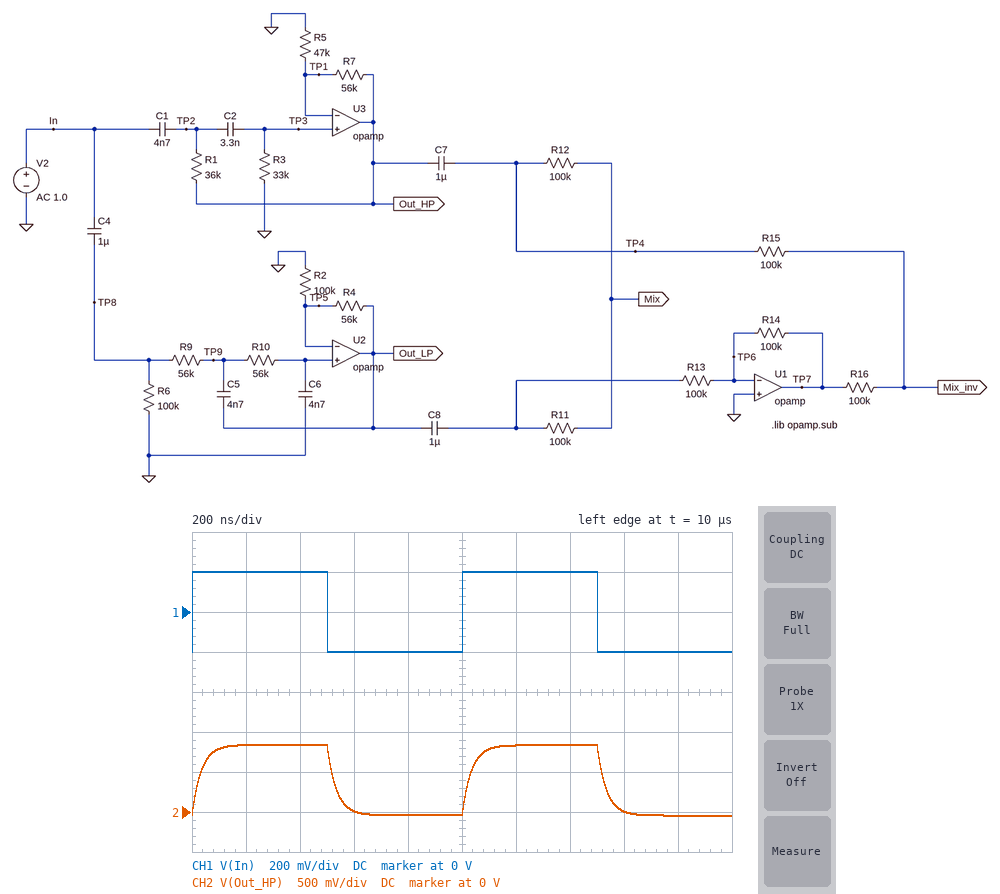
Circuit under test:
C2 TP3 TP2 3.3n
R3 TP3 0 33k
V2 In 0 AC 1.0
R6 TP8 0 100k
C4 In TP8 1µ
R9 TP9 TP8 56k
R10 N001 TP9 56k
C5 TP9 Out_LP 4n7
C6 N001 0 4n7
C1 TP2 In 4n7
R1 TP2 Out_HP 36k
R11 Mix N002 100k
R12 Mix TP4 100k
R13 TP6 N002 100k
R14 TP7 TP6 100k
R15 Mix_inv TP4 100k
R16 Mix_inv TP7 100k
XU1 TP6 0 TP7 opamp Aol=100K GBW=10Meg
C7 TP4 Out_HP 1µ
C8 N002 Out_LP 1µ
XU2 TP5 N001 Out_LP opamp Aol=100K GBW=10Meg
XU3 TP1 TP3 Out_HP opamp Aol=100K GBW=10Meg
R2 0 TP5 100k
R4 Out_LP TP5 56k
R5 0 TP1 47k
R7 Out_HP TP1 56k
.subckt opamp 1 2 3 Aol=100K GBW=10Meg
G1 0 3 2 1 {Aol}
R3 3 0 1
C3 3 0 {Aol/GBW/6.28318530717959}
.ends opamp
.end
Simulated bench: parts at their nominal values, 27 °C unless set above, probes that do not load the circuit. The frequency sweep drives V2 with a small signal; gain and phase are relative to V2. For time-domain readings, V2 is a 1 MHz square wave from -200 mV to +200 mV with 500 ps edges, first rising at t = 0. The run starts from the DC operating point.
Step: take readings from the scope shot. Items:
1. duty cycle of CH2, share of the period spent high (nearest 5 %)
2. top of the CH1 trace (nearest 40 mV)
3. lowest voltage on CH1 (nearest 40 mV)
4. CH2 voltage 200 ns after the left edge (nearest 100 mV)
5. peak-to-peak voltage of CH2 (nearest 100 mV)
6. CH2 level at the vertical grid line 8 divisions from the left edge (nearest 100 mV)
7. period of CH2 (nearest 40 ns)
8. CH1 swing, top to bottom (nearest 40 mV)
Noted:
50 %
200 mV
-200 mV
800 mV
900 mV
0 V
1.00 µs
400 mV
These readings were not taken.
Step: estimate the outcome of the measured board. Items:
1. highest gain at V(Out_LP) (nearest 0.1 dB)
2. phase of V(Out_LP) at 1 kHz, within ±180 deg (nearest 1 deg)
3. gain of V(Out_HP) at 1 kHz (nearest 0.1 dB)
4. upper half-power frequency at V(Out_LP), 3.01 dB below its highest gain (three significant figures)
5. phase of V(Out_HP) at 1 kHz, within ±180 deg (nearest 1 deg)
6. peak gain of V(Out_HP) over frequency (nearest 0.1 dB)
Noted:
3.8 dB
-126 deg
3.8 dB
593 Hz
105 deg
7.3 dB
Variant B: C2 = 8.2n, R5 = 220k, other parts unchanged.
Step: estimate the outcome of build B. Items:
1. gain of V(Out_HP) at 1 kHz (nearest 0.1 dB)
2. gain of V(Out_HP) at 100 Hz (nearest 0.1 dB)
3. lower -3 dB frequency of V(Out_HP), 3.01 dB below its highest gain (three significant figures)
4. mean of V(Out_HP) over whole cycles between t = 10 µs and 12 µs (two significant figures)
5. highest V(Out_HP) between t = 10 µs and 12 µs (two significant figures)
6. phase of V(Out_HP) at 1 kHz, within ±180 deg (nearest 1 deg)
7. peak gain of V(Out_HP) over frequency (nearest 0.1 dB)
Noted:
-1.2 dB
-33.0 dB
1.03 kHz
230 mV
480 mV
72 deg
2.0 dB
